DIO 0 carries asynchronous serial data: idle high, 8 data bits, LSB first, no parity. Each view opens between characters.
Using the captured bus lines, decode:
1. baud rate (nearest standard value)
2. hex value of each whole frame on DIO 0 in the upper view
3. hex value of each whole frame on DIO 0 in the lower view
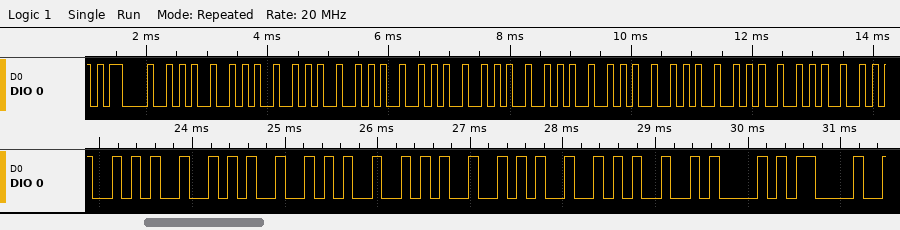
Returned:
9600 baud
0D, 2A, 2A, 2A, 2A, 2A, 2A, 2A, 2A, 2A, 2A, 2A
2A, 2A, 2A, 2A, 2A, 2A, 0A, 0D
